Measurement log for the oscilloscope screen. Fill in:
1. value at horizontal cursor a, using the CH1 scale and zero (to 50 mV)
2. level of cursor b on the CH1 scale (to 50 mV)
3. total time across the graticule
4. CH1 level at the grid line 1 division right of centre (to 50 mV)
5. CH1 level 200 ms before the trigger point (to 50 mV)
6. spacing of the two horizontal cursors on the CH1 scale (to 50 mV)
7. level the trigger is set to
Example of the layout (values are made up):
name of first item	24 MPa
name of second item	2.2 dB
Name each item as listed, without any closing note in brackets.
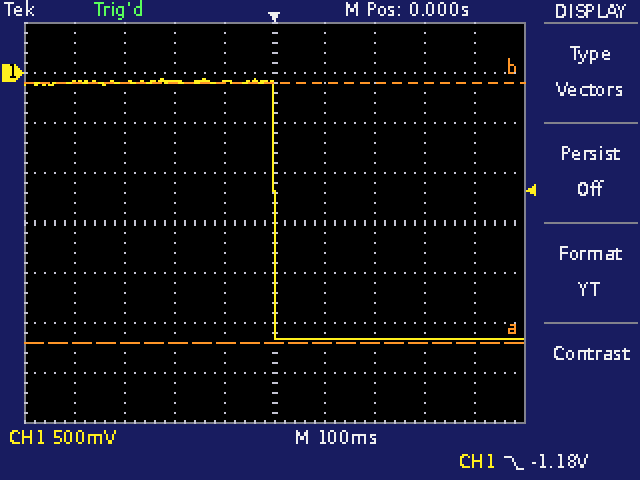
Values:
value at horizontal cursor a, using the CH1 scale and zero	-2.70 V
level of cursor b on the CH1 scale	-100 mV
total time across the graticule	1 s
CH1 level at the grid line 1 division right of centre	-2.65 V
CH1 level 200 ms before the trigger point	-100 mV
spacing of the two horizontal cursors on the CH1 scale	2.60 V
level the trigger is set to	-1.18 V
